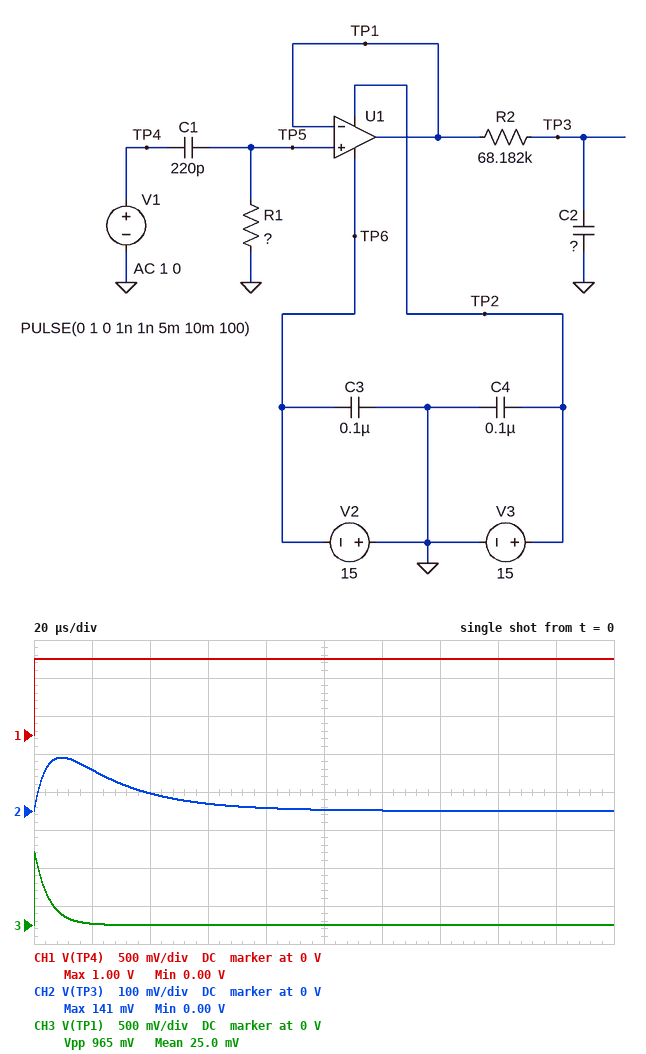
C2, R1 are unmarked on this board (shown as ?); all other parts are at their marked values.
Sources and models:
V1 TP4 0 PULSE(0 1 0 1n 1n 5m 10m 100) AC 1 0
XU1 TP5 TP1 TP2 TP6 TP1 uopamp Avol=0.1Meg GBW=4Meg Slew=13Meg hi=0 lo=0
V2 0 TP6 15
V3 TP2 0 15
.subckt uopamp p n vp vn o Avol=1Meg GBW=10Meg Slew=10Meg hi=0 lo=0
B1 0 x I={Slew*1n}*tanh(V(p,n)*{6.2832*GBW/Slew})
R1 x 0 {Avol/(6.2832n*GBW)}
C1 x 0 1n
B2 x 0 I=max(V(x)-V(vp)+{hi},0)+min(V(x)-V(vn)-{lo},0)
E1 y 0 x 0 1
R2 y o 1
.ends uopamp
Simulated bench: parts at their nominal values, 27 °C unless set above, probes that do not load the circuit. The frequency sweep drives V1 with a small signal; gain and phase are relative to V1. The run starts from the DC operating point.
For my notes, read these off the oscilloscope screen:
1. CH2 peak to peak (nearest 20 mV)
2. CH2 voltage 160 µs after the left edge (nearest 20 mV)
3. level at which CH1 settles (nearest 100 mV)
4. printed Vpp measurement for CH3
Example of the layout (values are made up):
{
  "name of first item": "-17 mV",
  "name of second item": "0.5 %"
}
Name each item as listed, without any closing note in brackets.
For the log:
{
  "CH2 peak to peak": "140 mV",
  "CH2 voltage 160 µs after the left edge": "0 V",
  "level at which CH1 settles": "1.0 V",
  "printed Vpp measurement for CH3": "965 mV"
}
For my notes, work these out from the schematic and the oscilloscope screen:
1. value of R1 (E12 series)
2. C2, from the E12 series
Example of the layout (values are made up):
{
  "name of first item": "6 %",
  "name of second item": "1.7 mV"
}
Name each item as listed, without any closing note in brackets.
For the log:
{
  "value of R1": "22 kΩ",
  "C2, from the E12 series": "330 pF"
}
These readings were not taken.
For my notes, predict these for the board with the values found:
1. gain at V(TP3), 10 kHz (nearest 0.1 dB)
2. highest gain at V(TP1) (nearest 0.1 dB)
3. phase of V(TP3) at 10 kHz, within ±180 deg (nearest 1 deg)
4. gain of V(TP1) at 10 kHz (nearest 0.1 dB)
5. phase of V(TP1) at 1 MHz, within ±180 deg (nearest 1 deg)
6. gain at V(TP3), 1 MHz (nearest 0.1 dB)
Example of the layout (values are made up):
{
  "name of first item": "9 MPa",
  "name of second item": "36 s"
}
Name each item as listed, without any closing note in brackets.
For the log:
{
  "gain at V(TP3), 10 kHz": "-15.5 dB",
  "highest gain at V(TP1)": "-0.1 dB",
  "phase of V(TP3) at 10 kHz, within ±180 deg": "18 deg",
  "gain of V(TP1) at 10 kHz": "-10.7 dB",
  "phase of V(TP1) at 1 MHz, within ±180 deg": "-12 deg",
  "gain at V(TP3), 1 MHz": "-43.3 dB"
}
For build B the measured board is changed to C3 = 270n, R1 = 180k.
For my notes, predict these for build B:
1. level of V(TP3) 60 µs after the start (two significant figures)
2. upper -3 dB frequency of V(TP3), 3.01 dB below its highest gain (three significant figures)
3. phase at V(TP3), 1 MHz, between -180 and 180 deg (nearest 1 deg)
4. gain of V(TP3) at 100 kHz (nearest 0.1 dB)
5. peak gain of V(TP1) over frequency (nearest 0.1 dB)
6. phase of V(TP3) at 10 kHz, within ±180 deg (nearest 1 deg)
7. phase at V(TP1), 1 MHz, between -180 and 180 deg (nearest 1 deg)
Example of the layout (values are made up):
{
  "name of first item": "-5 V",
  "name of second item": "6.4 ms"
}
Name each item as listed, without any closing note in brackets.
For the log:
{
  "level of V(TP3) 60 µs after the start": "350 mV",
  "upper -3 dB frequency of V(TP3), 3.01 dB below its highest gain": "13.2 kHz",
  "phase at V(TP3), 1 MHz, between -180 and 180 deg": "-103 deg",
  "gain of V(TP3) at 100 kHz": "-23.0 dB",
  "peak gain of V(TP1) over frequency": "0 dB",
  "phase of V(TP3) at 10 kHz, within ±180 deg": "-33 deg",
  "phase at V(TP1), 1 MHz, between -180 and 180 deg": "-14 deg"
}
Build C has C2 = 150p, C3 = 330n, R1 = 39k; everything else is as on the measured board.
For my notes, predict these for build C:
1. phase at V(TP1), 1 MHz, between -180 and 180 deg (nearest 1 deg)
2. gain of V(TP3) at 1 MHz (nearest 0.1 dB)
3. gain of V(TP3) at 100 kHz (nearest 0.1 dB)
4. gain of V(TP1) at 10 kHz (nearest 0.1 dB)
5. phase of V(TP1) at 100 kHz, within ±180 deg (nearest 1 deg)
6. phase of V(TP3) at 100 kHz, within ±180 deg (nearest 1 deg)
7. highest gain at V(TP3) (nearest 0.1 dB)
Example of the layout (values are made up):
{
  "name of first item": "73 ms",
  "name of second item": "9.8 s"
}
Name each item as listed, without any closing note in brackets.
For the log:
{
  "phase at V(TP1), 1 MHz, between -180 and 180 deg": "-13 deg",
  "gain of V(TP3) at 1 MHz": "-36.4 dB",
  "gain of V(TP3) at 100 kHz": "-16.4 dB",
  "gain of V(TP1) at 10 kHz": "-6.5 dB",
  "phase of V(TP1) at 100 kHz, within ±180 deg": "9 deg",
  "phase of V(TP3) at 100 kHz, within ±180 deg": "-72 deg",
  "highest gain at V(TP3)": "-6.8 dB"
}
